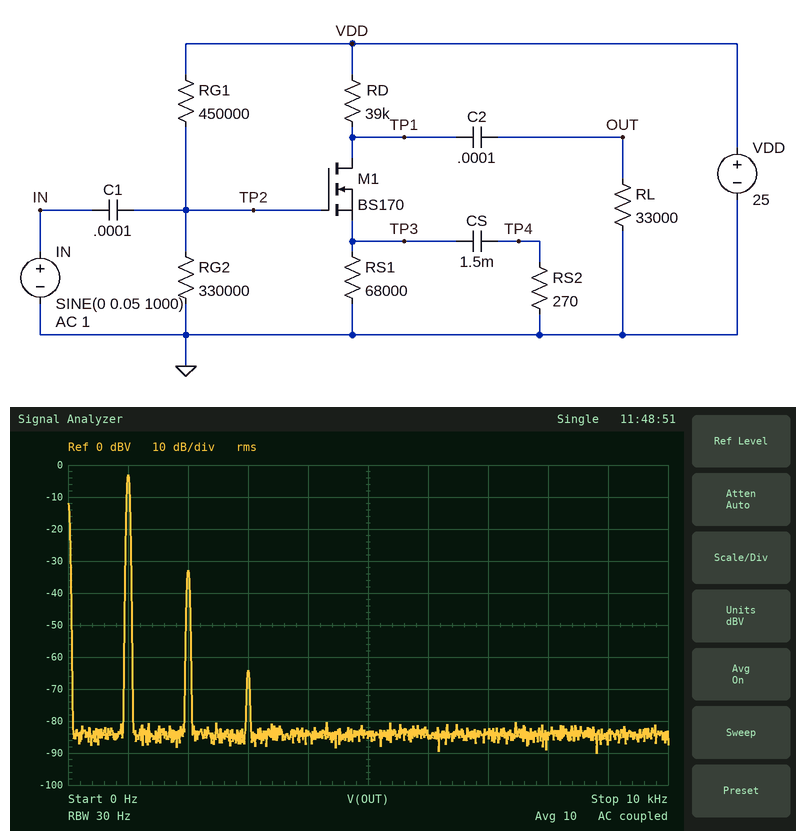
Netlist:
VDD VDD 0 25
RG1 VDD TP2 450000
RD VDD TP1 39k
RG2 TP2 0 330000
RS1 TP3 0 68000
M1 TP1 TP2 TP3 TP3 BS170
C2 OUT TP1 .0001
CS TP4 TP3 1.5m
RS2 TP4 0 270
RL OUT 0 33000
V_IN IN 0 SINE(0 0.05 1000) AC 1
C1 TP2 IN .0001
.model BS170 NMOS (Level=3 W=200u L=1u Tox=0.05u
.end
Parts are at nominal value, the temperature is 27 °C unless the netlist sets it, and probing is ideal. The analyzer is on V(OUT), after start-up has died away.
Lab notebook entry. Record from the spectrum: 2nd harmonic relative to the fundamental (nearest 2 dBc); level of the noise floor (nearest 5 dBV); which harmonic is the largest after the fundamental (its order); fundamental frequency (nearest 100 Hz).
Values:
-30 dBc
-85 dBV
2
1.0 kHz
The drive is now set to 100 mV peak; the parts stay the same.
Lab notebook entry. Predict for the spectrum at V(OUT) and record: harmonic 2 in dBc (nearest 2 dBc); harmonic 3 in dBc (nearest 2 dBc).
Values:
-24 dBc
-48 dBc
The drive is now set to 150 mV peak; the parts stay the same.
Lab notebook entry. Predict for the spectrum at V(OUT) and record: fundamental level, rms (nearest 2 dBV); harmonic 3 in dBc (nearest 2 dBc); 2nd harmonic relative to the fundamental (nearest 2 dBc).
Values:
6 dBV
-42 dBc
-20 dBc
